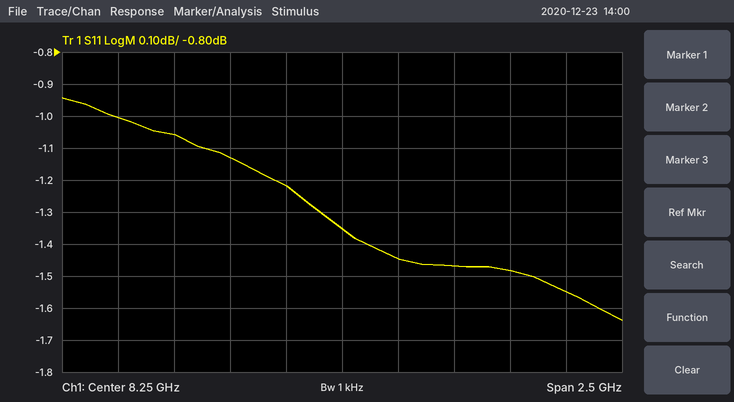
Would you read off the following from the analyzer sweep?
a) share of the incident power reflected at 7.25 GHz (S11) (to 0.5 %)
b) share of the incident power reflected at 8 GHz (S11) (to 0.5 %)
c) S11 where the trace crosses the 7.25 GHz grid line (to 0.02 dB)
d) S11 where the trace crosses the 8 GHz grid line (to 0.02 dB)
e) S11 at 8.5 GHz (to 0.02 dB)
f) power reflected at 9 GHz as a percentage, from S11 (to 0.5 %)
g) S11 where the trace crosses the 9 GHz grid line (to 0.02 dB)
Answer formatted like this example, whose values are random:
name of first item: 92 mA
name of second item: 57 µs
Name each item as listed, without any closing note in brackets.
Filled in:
share of the incident power reflected at 7.25 GHz (S11): 79.5 %
share of the incident power reflected at 8 GHz (S11): 75.5 %
S11 where the trace crosses the 7.25 GHz grid line: -1.00 dB
S11 where the trace crosses the 8 GHz grid line: -1.22 dB
S11 at 8.5 GHz: -1.44 dB
power reflected at 9 GHz as a percentage, from S11: 71.0 %
S11 where the trace crosses the 9 GHz grid line: -1.48 dB
